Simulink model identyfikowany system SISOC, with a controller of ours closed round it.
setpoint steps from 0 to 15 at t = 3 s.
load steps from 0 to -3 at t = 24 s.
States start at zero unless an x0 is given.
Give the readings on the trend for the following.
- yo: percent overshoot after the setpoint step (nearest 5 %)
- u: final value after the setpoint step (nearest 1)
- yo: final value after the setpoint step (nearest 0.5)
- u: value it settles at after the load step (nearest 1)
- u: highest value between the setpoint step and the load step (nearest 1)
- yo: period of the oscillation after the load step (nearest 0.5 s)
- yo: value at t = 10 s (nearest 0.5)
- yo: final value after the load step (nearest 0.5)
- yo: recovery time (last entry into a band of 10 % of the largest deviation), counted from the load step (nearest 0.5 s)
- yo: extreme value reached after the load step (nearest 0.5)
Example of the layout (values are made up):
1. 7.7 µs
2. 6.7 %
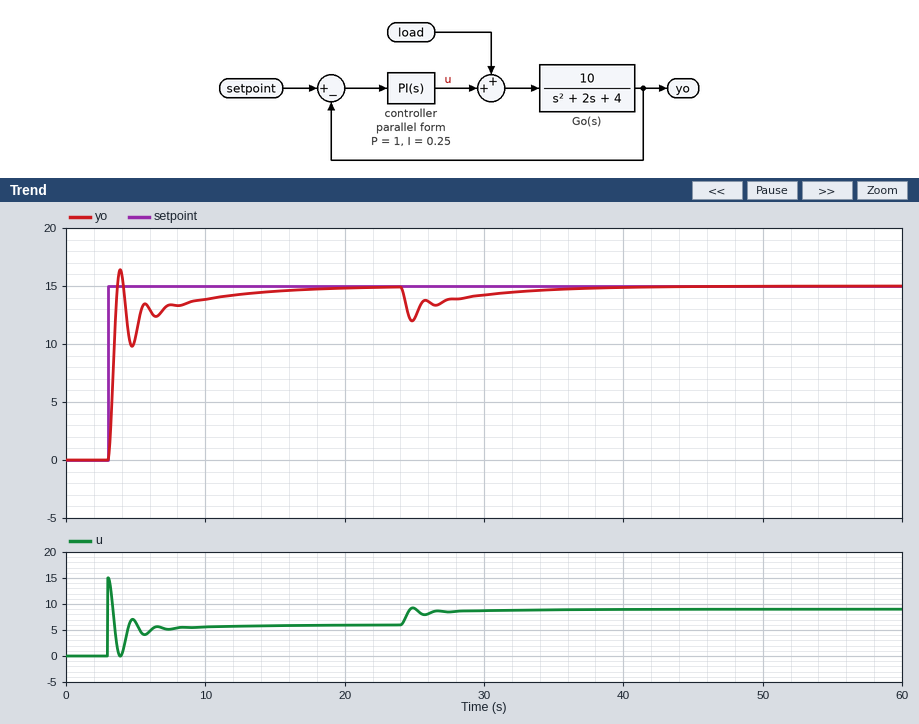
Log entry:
1. 10 %
2. 6
3. 15.0
4. 9
5. 15
6. 1.5 s
7. 14.0
8. 15.0
9. 11.5 s
10. 12.0
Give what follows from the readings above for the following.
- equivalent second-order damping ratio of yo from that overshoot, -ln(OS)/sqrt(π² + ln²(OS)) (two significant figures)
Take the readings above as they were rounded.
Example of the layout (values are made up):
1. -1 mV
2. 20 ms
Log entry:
1. 0.59
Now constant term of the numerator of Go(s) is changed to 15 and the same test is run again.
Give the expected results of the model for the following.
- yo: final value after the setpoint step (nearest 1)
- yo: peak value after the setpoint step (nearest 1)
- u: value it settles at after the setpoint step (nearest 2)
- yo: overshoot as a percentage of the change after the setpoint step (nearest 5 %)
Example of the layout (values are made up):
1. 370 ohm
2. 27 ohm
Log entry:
1. 15
2. 19
3. 4
4. 25 %
